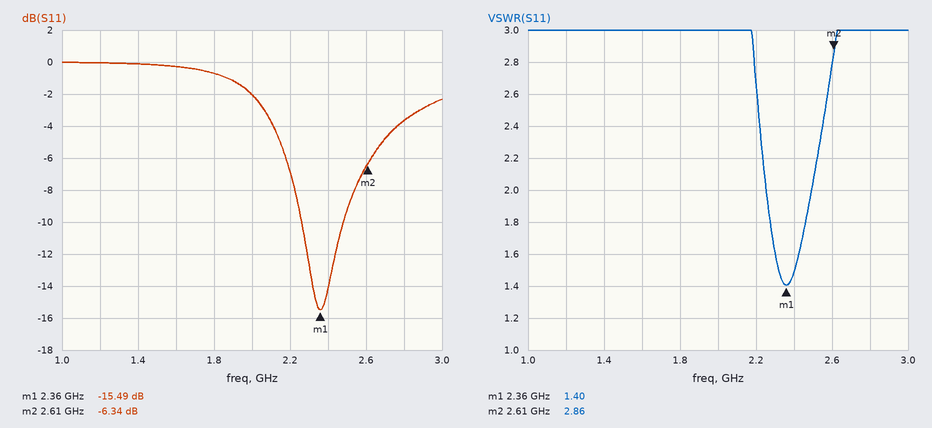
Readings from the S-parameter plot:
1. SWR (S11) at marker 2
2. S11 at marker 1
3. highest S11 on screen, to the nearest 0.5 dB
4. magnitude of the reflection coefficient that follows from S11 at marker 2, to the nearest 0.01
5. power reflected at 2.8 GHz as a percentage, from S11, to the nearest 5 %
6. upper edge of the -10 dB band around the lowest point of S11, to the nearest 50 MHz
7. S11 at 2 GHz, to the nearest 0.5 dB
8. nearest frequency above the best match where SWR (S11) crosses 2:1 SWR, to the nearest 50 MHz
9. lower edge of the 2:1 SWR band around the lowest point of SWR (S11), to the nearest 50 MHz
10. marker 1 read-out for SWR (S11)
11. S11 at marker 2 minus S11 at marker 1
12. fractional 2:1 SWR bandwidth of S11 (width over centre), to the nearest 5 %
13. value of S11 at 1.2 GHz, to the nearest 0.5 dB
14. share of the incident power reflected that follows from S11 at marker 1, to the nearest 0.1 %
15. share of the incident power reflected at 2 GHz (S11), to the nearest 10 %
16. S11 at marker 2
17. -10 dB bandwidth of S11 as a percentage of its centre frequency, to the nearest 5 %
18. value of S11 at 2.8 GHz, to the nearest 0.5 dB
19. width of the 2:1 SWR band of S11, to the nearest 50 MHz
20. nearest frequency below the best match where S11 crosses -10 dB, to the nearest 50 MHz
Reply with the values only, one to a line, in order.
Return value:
2.86
-15.49 dB
0.0 dB
0.48
45 %
2.50 GHz
-2.0 dB
2.50 GHz
2.25 GHz
1.40
9.15 dB
10 %
0.0 dB
2.8 %
60 %
-6.34 dB
10 %
-3.5 dB
250 MHz
2.25 GHz
